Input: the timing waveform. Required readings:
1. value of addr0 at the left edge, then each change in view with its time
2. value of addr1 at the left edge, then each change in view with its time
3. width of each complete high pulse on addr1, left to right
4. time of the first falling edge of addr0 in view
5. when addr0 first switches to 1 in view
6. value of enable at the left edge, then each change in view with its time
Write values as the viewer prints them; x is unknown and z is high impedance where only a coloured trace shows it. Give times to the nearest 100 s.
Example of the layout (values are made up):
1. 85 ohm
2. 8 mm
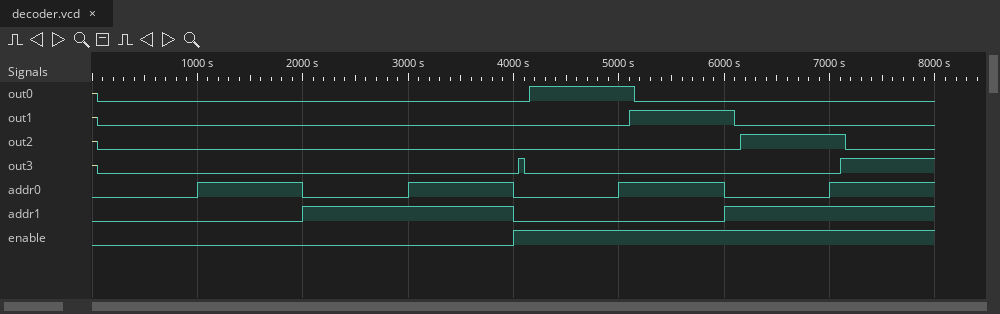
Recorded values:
1. 0, 1 at 1000 s, 0 at 2000 s, 1 at 3000 s, 0 at 4000 s, 1 at 5000 s, 0 at 6000 s, 1 at 7000 s
2. 0, 1 at 2000 s, 0 at 4000 s, 1 at 6000 s
3. 2000 s
4. 2000 s
5. 1000 s
6. 0, 1 at 4000 s
